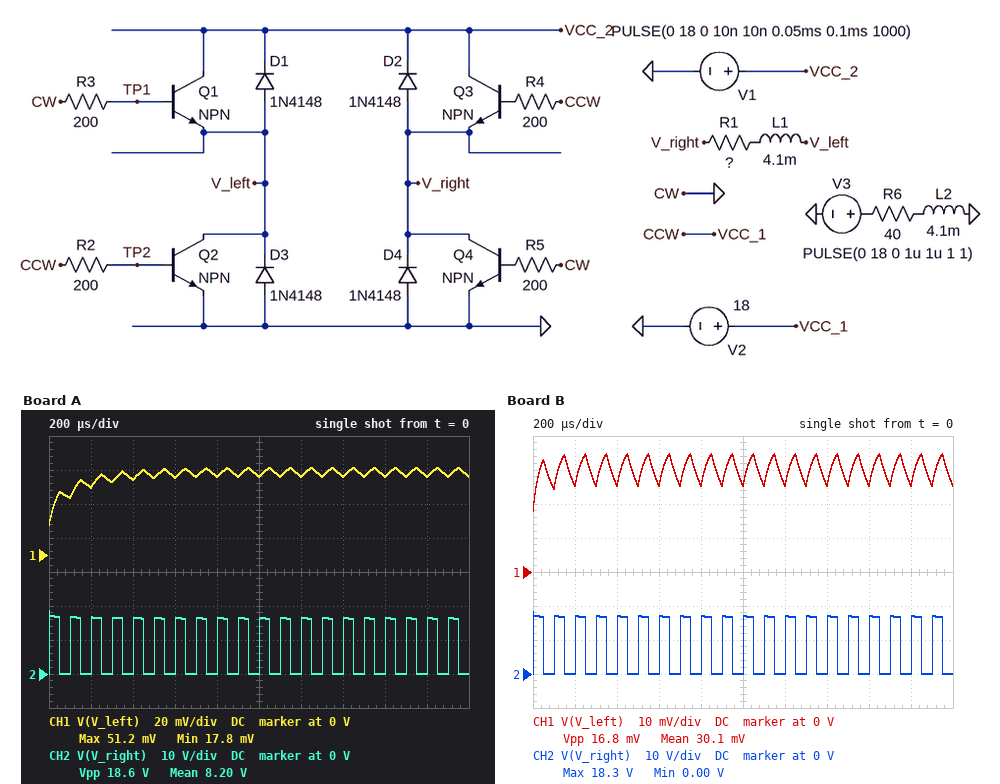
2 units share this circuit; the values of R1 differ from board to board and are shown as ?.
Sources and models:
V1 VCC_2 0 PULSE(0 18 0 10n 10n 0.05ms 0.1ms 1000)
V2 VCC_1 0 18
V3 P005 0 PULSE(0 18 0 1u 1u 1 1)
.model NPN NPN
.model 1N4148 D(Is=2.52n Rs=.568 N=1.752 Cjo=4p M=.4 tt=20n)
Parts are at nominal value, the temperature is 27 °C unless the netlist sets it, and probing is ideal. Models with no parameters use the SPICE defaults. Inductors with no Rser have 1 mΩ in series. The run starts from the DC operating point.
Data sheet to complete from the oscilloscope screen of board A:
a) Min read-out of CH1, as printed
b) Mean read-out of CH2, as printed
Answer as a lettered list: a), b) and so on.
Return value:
a) 17.8 mV
b) 8.20 V
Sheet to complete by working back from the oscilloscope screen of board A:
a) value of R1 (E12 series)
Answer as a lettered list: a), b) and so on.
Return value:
a) 22 Ω
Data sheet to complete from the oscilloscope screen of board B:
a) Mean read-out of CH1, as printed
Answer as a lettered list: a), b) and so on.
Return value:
a) 30.1 mV
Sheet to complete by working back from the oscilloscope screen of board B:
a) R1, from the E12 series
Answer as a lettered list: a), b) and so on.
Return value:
a) 82 Ω
